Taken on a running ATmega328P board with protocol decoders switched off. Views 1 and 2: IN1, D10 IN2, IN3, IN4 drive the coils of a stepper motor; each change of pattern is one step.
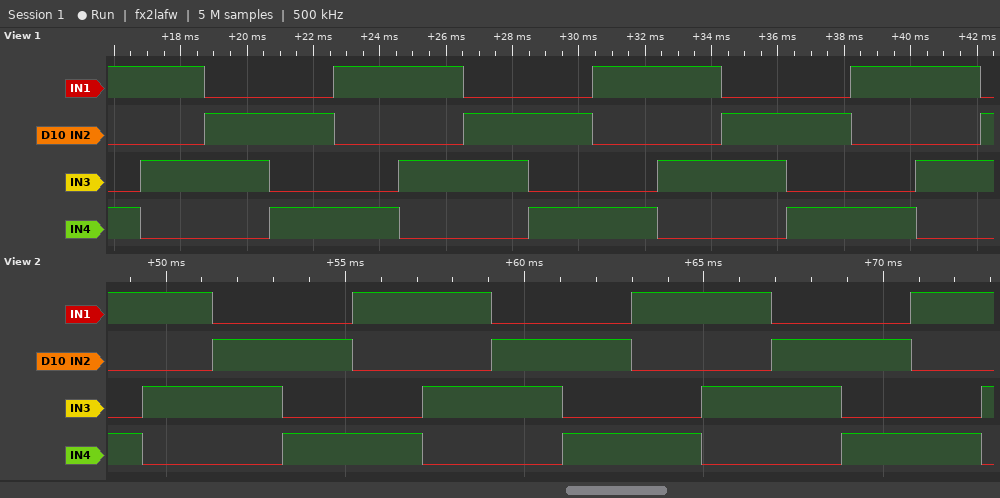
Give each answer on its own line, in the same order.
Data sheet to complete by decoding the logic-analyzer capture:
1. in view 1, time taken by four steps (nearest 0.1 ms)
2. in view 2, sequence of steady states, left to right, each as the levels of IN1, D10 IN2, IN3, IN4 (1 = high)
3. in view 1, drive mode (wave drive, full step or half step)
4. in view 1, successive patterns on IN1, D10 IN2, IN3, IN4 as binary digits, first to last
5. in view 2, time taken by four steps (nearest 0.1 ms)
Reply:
7.8 ms
1001 1010 0110 0101 1001 1010 0110 0101 1001 1010 0110 0101 1001 1010
full step
1001 1010 0110 0101 1001 1010 0110 0101 1001 1010 0110 0101 1001 1010 0110
7.8 ms
